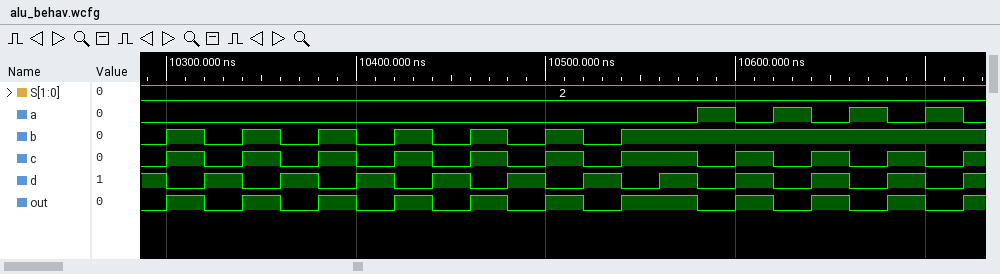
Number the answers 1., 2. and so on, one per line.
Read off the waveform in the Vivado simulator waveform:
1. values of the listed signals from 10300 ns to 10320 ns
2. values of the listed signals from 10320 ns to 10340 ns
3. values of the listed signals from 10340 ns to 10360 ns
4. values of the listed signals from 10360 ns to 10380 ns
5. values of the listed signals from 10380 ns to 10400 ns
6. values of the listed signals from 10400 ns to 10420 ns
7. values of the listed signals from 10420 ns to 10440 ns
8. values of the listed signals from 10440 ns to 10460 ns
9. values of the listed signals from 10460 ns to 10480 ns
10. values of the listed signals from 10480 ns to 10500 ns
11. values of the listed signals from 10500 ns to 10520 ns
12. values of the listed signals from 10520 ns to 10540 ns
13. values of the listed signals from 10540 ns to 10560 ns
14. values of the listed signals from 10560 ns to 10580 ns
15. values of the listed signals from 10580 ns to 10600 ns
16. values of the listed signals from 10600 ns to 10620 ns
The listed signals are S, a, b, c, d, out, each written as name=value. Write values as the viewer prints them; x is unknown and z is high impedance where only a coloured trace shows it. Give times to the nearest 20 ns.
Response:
1. S=2, a=0, b=1, c=1, d=0, out=1
2. S=2, a=0, b=0, c=0, d=1, out=0
3. S=2, a=0, b=1, c=1, d=0, out=1
4. S=2, a=0, b=0, c=0, d=1, out=0
5. S=2, a=0, b=1, c=1, d=0, out=1
6. S=2, a=0, b=0, c=0, d=1, out=0
7. S=2, a=0, b=1, c=1, d=0, out=1
8. S=2, a=0, b=0, c=0, d=1, out=0
9. S=2, a=0, b=1, c=1, d=0, out=1
10. S=2, a=0, b=0, c=0, d=1, out=0
11. S=2, a=0, b=1, c=1, d=0, out=1
12. S=2, a=0, b=0, c=0, d=1, out=0
13. S=2, a=0, b=1, c=1, d=0, out=1
14. S=2, a=0, b=1, c=1, d=1, out=1
15. S=2, a=1, b=1, c=0, d=0, out=0
16. S=2, a=0, b=1, c=1, d=1, out=1
